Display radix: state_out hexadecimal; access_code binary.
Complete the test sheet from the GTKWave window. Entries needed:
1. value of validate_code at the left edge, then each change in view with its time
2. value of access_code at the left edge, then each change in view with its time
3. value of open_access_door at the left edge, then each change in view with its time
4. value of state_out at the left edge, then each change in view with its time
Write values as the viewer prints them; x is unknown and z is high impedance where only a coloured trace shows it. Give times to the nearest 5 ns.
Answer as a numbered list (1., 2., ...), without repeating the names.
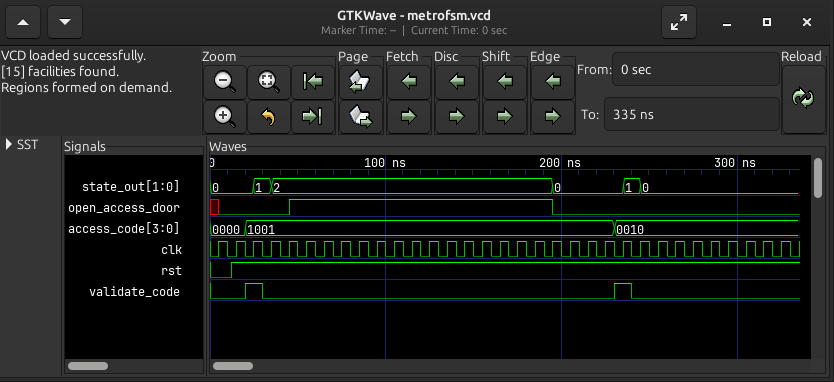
1. 0, 1 at 20 ns, 0 at 30 ns, 1 at 230 ns, 0 at 240 ns
2. 0000, 1001 at 20 ns, 0010 at 230 ns
3. x, 0 at 5 ns, 1 at 45 ns, 0 at 195 ns
4. 0, 1 at 25 ns, 2 at 35 ns, 0 at 195 ns, 1 at 235 ns, 0 at 245 ns
